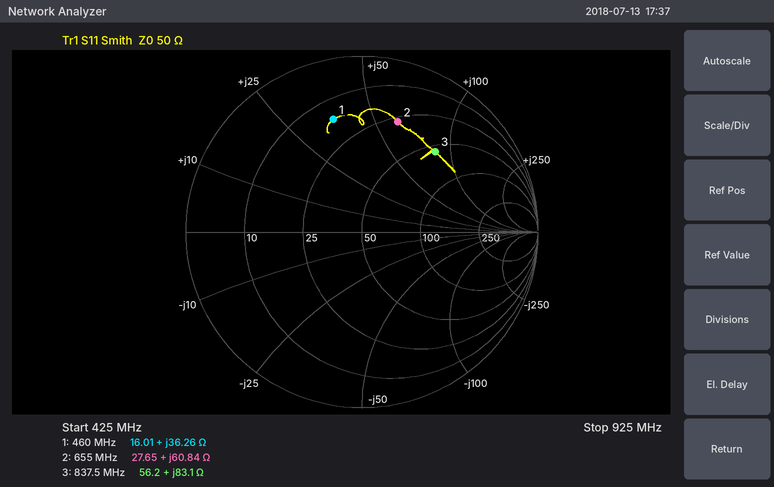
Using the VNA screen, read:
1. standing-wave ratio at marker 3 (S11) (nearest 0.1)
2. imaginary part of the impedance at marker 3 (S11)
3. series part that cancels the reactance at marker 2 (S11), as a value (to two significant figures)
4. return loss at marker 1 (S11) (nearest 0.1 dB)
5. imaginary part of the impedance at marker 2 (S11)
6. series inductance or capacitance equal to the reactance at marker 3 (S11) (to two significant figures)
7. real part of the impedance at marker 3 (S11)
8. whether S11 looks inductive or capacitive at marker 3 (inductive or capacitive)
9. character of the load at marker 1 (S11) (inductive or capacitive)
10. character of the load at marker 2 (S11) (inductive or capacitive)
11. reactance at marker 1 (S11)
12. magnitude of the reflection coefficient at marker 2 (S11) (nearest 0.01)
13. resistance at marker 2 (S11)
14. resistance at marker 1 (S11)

4.2
+83.1 Ω
4.0 pF
3.6 dB
+60.84 Ω
16 nH
56.2 Ω
inductive
inductive
inductive
+36.26 Ω
0.66
27.65 Ω
16.01 Ω
